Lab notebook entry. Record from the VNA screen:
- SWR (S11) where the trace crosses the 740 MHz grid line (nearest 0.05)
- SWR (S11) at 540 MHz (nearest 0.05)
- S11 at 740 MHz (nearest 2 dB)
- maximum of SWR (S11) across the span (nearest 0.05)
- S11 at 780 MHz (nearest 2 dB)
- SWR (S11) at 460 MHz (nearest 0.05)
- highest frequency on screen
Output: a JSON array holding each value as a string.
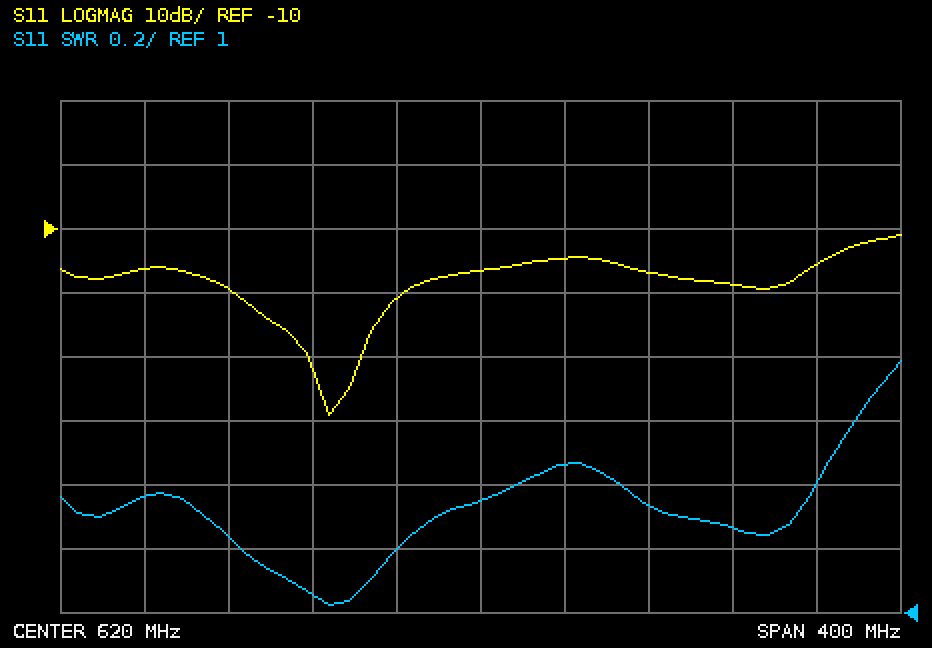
["1.25", "1.05", "-18 dB", "1.80", "-16 dB", "1.35", "820 MHz"]
